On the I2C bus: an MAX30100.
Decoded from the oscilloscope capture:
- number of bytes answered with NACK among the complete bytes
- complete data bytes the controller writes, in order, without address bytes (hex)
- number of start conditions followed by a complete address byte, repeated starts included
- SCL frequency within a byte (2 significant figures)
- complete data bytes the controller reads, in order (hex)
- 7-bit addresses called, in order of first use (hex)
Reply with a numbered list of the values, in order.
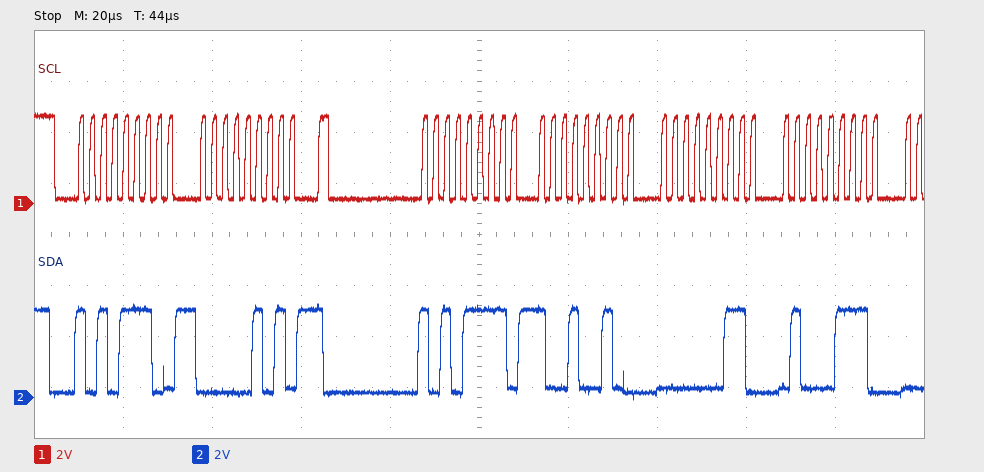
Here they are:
1. 0
2. 05
3. 2
4. 400 kHz
5. 92 03 47
6. 0x57
